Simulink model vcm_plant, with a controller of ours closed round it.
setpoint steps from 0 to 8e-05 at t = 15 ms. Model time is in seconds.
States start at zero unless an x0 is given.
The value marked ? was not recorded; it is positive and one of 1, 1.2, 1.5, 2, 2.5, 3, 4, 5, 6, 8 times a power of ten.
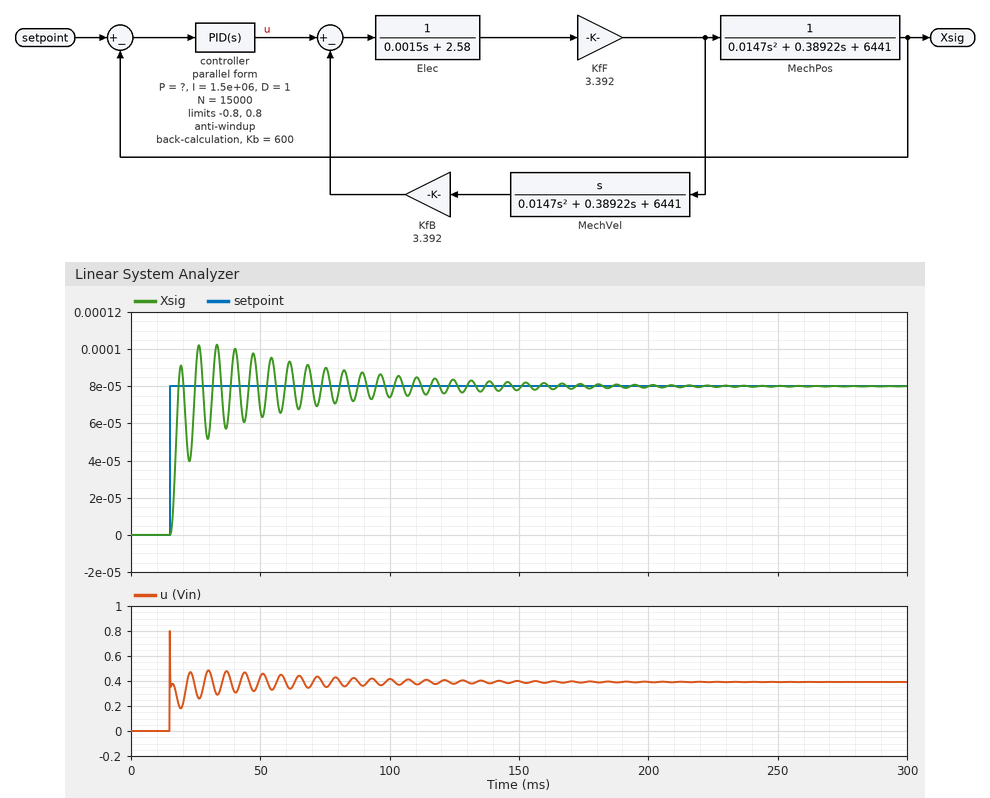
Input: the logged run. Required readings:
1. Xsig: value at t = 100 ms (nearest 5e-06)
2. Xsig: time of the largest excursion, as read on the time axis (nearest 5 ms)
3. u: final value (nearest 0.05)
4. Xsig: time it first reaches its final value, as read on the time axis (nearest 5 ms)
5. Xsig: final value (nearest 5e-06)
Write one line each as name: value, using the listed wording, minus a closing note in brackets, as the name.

Xsig: value at t = 100 ms: 0.000075
Xsig: time of the largest excursion, as read on the time axis: 35 ms
u: final value: 0.40
Xsig: time it first reaches its final value, as read on the time axis: 20 ms
Xsig: final value: 0.000080
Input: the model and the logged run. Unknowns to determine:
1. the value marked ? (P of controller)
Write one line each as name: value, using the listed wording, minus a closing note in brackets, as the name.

the value marked ?: 4000
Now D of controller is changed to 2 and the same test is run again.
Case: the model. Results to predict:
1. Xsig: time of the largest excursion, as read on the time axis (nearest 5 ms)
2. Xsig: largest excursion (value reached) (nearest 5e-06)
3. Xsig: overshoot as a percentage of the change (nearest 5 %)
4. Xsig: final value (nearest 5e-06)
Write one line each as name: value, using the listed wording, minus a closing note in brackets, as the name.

Xsig: time of the largest excursion, as read on the time axis: 25 ms
Xsig: largest excursion (value reached): 0.000090
Xsig: overshoot as a percentage of the change: 10 %
Xsig: final value: 0.000080
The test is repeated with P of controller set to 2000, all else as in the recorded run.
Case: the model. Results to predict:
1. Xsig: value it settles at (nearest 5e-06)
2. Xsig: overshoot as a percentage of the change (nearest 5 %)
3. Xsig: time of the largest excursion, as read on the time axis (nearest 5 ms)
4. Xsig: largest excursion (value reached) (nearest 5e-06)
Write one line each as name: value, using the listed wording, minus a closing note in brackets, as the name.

Xsig: value it settles at: 0.000080
Xsig: overshoot as a percentage of the change: 15 %
Xsig: time of the largest excursion, as read on the time axis: 30 ms
Xsig: largest excursion (value reached): 0.000090
